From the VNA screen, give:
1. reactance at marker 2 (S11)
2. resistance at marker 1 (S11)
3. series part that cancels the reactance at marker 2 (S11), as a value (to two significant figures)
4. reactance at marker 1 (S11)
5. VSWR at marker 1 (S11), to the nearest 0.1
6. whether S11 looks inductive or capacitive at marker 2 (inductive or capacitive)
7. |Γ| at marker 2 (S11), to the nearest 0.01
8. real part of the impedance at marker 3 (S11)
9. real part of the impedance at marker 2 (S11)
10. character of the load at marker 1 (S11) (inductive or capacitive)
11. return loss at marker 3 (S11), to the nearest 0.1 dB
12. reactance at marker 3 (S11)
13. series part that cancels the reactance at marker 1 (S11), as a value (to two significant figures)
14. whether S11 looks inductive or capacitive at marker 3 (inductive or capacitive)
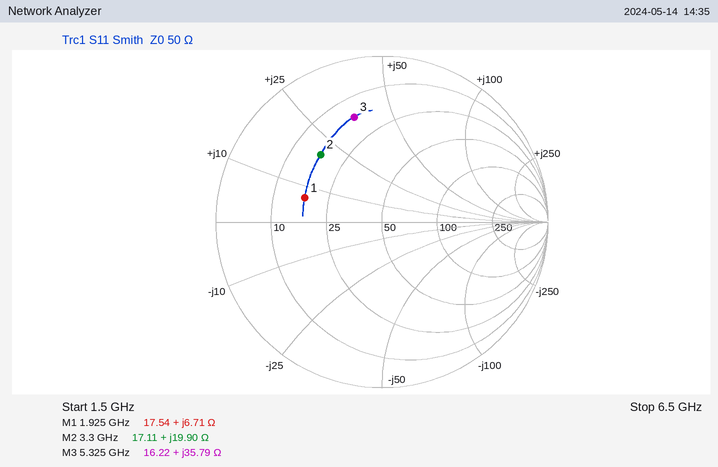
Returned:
+19.90 Ω
17.54 Ω
2.4 pF
+6.71 Ω
2.9
inductive
0.55
16.22 Ω
17.11 Ω
inductive
3.7 dB
+35.79 Ω
12 pF
inductive
